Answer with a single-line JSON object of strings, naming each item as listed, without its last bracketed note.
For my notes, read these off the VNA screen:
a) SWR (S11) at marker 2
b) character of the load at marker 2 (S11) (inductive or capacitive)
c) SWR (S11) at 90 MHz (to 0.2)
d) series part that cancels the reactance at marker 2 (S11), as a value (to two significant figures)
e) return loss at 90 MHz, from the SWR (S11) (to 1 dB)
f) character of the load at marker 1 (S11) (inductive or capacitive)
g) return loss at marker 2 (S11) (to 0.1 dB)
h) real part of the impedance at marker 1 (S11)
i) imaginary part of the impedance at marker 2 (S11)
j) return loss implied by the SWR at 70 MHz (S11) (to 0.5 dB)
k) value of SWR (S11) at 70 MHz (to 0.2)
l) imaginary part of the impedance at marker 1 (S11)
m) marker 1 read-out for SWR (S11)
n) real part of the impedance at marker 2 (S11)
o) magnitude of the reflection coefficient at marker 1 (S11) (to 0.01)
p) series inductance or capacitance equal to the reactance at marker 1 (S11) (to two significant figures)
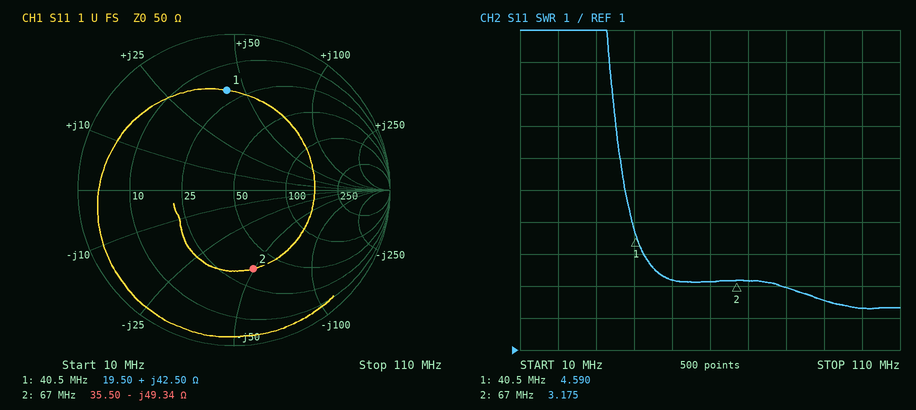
{"SWR (S11) at marker 2": "3.175", "character of the load at marker 2 (S11)": "capacitive", "SWR (S11) at 90 MHz": "2.6", "series part that cancels the reactance at marker 2 (S11), as a value": "120 nH", "return loss at 90 MHz, from the SWR (S11)": "7 dB", "character of the load at marker 1 (S11)": "inductive", "return loss at marker 2 (S11)": "5.7 dB", "real part of the impedance at marker 1": "19.50 Ω", "imaginary part of the impedance at marker 2": "-49.34 Ω", "return loss implied by the SWR at 70 MHz (S11)": "5.5 dB", "value of SWR (S11) at 70 MHz": "3.2", "imaginary part of the impedance at marker 1": "+42.50 Ω", "marker 1 read-out for SWR": "4.590", "real part of the impedance at marker 2": "35.50 Ω", "magnitude of the reflection coefficient at marker 1 (S11)": "0.64", "series inductance or capacitance equal to the reactance at marker 1 (S11)": "170 nH"}
